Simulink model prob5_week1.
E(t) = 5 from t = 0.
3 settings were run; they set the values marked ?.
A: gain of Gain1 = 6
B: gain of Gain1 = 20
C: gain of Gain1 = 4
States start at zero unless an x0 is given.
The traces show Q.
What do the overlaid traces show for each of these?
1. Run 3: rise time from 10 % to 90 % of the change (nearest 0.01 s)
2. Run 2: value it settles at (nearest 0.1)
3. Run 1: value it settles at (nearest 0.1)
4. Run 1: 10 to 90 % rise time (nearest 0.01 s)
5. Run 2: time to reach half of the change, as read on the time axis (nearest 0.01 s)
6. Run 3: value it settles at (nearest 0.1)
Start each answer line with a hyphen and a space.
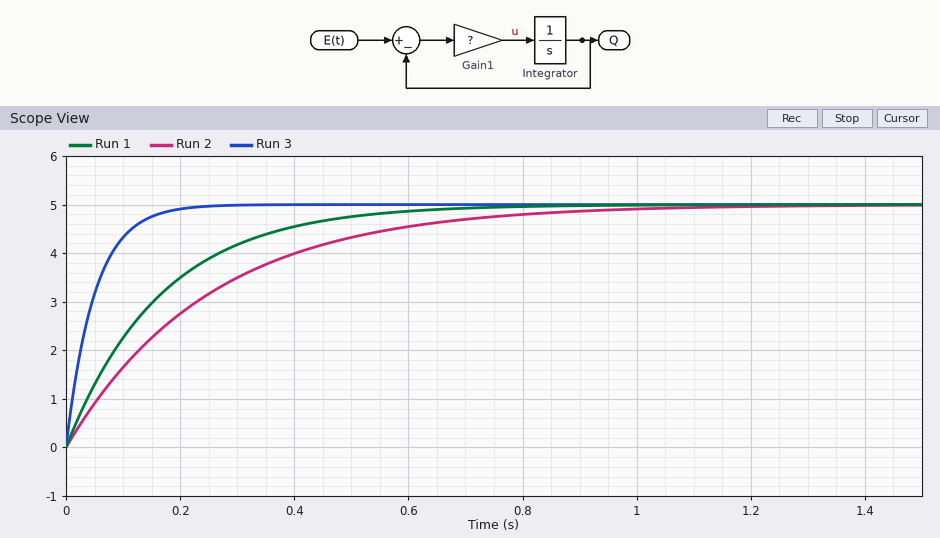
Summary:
- 0.11 s
- 5.0
- 5.0
- 0.37 s
- 0.17 s
- 5.0
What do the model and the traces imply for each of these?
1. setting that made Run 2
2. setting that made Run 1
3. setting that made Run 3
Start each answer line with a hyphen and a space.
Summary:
- C
- A
- B
